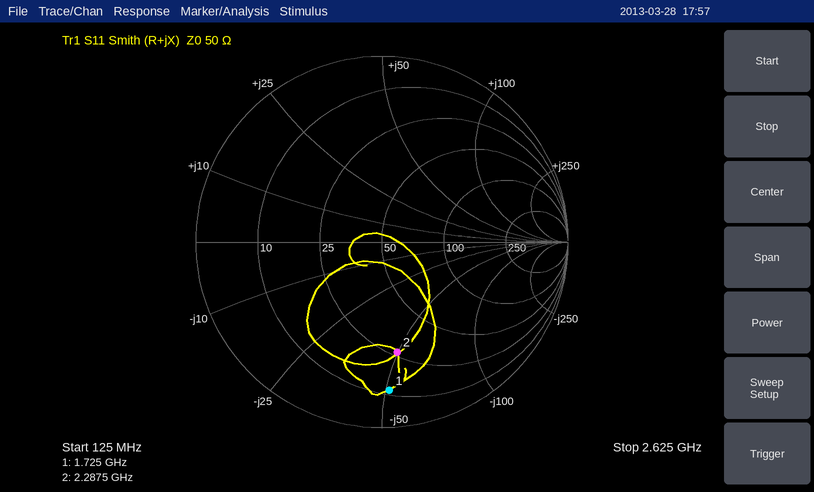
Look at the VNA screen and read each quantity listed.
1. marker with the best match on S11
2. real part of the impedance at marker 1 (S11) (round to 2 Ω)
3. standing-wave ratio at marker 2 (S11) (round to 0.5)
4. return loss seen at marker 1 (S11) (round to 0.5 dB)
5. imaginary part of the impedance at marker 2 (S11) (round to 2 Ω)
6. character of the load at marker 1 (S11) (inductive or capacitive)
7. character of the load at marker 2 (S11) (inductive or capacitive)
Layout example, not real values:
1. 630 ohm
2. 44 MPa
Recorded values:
1. marker 2
2. 12 Ω
3. 4.0
4. 2.0 dB
5. -50 Ω
6. capacitive
7. capacitive
